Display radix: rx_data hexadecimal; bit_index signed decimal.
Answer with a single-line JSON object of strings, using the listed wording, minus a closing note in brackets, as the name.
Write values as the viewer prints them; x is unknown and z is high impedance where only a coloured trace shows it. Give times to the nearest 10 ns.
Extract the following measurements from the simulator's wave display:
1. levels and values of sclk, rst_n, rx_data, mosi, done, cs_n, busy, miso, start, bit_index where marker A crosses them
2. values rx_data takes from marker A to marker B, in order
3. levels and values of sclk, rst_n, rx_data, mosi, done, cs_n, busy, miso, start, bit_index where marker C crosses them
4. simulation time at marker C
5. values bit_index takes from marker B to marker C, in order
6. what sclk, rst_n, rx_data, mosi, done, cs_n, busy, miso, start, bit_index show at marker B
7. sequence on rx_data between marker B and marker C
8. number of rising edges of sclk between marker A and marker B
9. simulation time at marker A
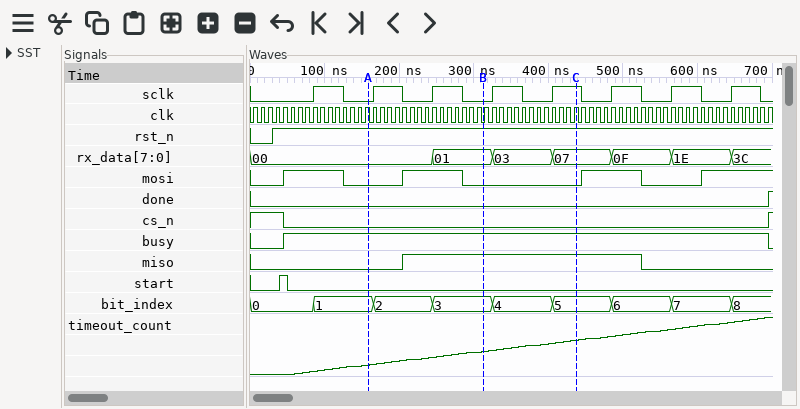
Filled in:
{"levels and values of sclk, rst_n, rx_data, mosi, done, cs_n, busy, miso, start, bit_index where marker A crosses them": "sclk=0, rst_n=1, rx_data=00, mosi=0, done=0, cs_n=0, busy=1, miso=0, start=0, bit_index=1", "values rx_data takes from marker A to marker B, in order": "00, 01", "levels and values of sclk, rst_n, rx_data, mosi, done, cs_n, busy, miso, start, bit_index where marker C crosses them": "sclk=1, rst_n=1, rx_data=07, mosi=0, done=0, cs_n=0, busy=1, miso=1, start=0, bit_index=5", "simulation time at marker C": "440 ns", "values bit_index takes from marker B to marker C, in order": "3, 4, 5", "what sclk, rst_n, rx_data, mosi, done, cs_n, busy, miso, start, bit_index show at marker B": "sclk=0, rst_n=1, rx_data=01, mosi=0, done=0, cs_n=0, busy=1, miso=1, start=0, bit_index=3", "sequence on rx_data between marker B and marker C": "01, 03, 07", "number of rising edges of sclk between marker A and marker B": "2", "simulation time at marker A": "160 ns"}
